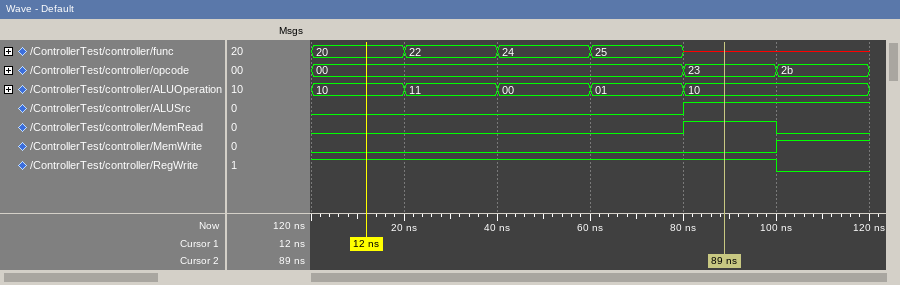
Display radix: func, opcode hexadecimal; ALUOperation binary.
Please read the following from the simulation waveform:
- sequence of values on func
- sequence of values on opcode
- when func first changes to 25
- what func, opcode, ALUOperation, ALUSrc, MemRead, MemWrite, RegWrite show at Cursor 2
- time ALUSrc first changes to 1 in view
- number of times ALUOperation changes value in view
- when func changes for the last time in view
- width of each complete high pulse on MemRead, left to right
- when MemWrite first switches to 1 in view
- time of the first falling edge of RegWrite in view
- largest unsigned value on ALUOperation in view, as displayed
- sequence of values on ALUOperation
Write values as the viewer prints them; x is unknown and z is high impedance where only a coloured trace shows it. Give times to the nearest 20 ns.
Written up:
20, 22, 24, 25, x
00, 23, 2b
60 ns
func=x, opcode=23, ALUOperation=10, ALUSrc=1, MemRead=1, MemWrite=0, RegWrite=1
80 ns
4
80 ns
20 ns
100 ns
100 ns
11
10, 11, 00, 01, 10
